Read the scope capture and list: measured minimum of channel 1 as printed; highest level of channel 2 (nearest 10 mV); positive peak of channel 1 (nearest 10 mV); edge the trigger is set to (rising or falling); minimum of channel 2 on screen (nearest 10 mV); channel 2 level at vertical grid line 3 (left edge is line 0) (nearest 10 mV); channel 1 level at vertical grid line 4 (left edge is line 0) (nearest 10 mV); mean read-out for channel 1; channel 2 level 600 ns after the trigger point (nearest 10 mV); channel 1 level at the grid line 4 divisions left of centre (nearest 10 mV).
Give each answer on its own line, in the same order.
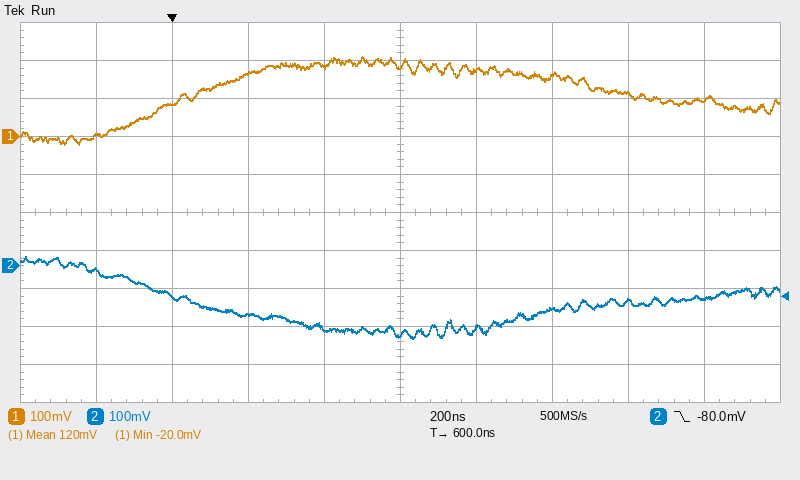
-20.0 mV
20 mV
210 mV
falling
-190 mV
-130 mV
190 mV
120 mV
-180 mV
0 mV
